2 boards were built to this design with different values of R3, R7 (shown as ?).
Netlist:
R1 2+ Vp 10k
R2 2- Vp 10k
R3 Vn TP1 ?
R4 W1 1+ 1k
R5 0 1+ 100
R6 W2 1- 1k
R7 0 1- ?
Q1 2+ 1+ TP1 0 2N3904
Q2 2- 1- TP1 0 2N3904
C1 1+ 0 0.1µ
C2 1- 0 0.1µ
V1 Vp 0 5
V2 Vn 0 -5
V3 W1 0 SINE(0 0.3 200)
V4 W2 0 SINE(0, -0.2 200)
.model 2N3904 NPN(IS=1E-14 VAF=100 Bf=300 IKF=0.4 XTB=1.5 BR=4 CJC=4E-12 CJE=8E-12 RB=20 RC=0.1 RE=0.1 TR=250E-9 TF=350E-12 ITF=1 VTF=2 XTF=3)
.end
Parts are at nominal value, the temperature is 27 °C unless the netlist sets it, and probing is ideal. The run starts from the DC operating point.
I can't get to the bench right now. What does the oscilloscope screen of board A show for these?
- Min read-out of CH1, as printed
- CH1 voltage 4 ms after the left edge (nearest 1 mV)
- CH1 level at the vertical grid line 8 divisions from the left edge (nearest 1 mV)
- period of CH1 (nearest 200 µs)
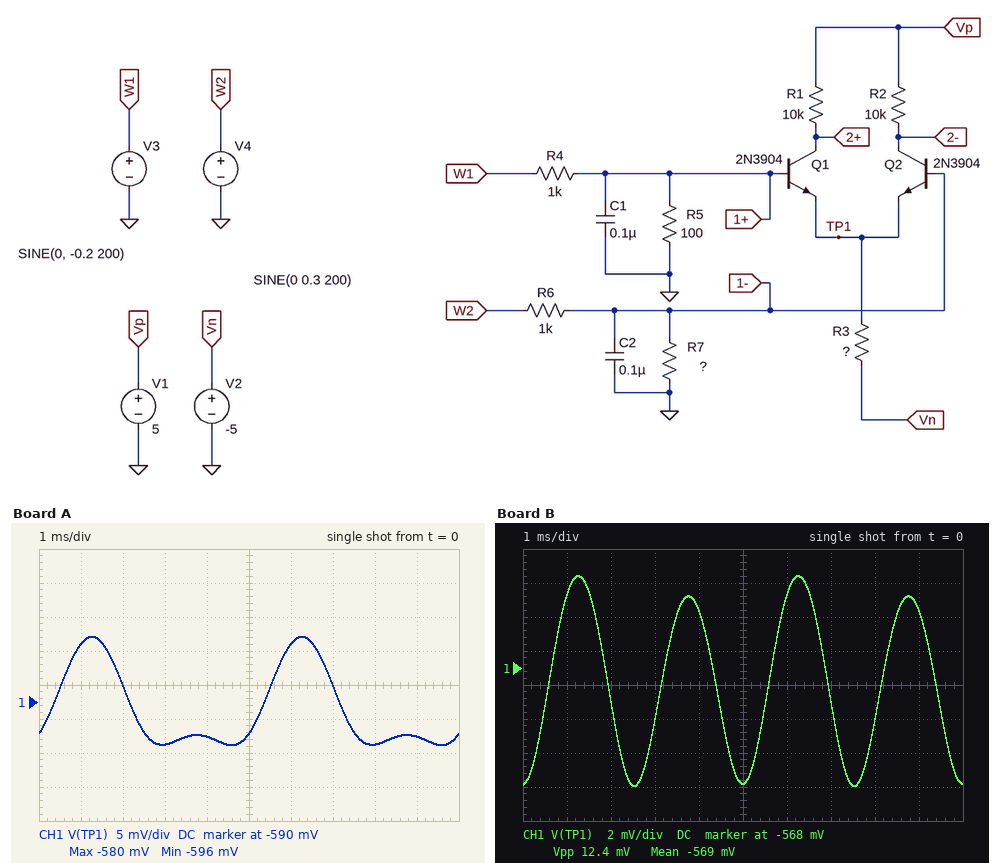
-596 mV
-595 mV
-596 mV
5.0 ms
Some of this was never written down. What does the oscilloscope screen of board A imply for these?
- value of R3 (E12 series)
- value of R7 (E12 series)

22 kΩ
68 Ω
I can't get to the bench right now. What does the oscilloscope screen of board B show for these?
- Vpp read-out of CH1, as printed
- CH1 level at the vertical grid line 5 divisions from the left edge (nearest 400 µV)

12.4 mV
-574.8 mV
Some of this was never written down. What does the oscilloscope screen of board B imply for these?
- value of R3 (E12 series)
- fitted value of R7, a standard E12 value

47 kΩ
150 Ω
